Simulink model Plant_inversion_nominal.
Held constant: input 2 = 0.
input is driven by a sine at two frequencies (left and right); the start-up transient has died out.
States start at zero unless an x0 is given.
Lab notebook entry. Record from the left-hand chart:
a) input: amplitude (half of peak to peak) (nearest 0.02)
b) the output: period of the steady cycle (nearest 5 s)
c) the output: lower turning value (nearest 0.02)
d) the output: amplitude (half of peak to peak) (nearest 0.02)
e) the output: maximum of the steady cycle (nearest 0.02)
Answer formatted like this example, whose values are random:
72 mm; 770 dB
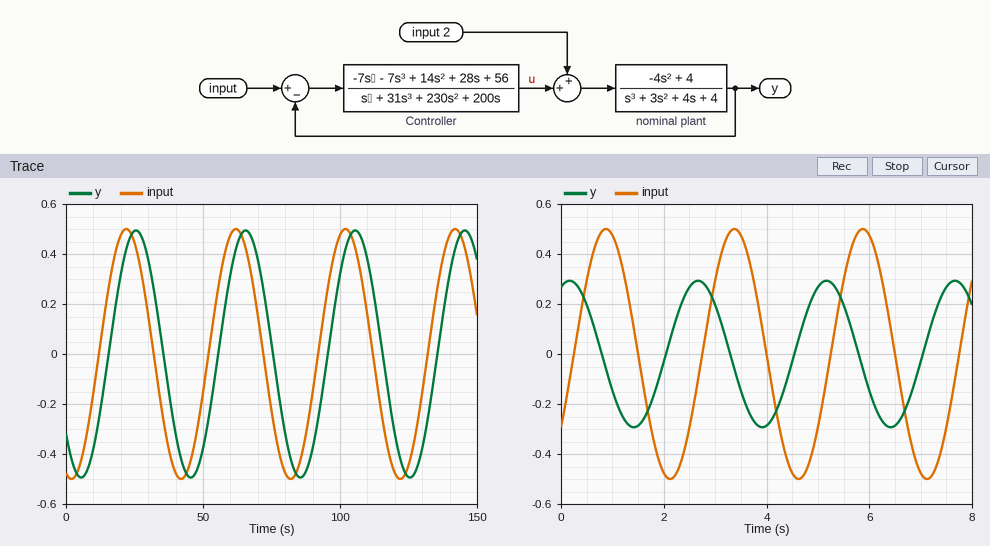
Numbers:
0.50; 40 s; -0.50; 0.50; 0.50
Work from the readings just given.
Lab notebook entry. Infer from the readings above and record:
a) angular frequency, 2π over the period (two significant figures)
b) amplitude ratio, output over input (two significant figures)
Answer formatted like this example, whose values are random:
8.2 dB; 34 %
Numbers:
0.16 rad/s; 1.0
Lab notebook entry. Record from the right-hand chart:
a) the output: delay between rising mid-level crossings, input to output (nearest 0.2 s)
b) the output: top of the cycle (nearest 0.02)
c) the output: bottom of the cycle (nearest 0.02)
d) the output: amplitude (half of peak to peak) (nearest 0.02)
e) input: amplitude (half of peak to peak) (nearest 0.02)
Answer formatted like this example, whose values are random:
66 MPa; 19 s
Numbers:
1.8 s; 0.30; -0.30; 0.30; 0.50
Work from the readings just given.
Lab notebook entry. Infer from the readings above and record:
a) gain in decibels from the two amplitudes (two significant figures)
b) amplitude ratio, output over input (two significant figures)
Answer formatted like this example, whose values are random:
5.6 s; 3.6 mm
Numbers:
-4.4 dB; 0.60
